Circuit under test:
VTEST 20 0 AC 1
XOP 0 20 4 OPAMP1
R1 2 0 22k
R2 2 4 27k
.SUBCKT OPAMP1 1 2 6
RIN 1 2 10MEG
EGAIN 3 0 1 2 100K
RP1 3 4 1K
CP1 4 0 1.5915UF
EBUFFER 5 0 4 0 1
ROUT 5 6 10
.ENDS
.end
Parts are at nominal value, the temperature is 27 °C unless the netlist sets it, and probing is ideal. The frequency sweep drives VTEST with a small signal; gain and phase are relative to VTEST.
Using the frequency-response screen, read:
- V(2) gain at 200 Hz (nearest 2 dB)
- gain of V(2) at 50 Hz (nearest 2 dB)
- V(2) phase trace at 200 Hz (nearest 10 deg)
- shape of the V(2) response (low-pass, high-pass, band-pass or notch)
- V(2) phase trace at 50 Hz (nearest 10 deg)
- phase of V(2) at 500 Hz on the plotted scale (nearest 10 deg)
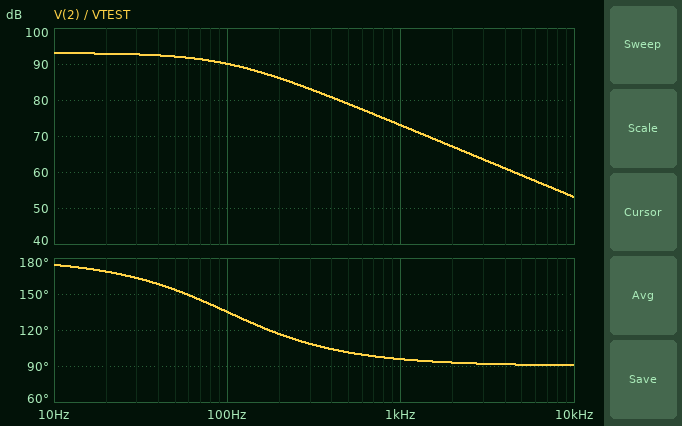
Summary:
86 dB
92 dB
120 deg
low-pass
150 deg
100 deg
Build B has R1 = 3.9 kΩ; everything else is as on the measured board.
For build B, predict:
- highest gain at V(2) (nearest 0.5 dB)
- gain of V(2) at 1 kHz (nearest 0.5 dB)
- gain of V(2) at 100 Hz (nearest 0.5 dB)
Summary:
82.0 dB
62.0 dB
79.0 dB
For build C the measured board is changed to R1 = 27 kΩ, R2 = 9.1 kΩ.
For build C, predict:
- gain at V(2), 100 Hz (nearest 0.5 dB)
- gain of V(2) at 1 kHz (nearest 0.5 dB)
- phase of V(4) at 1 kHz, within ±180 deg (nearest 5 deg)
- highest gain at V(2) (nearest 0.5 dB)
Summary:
94.5 dB
77.5 dB
95 deg
97.5 dB
